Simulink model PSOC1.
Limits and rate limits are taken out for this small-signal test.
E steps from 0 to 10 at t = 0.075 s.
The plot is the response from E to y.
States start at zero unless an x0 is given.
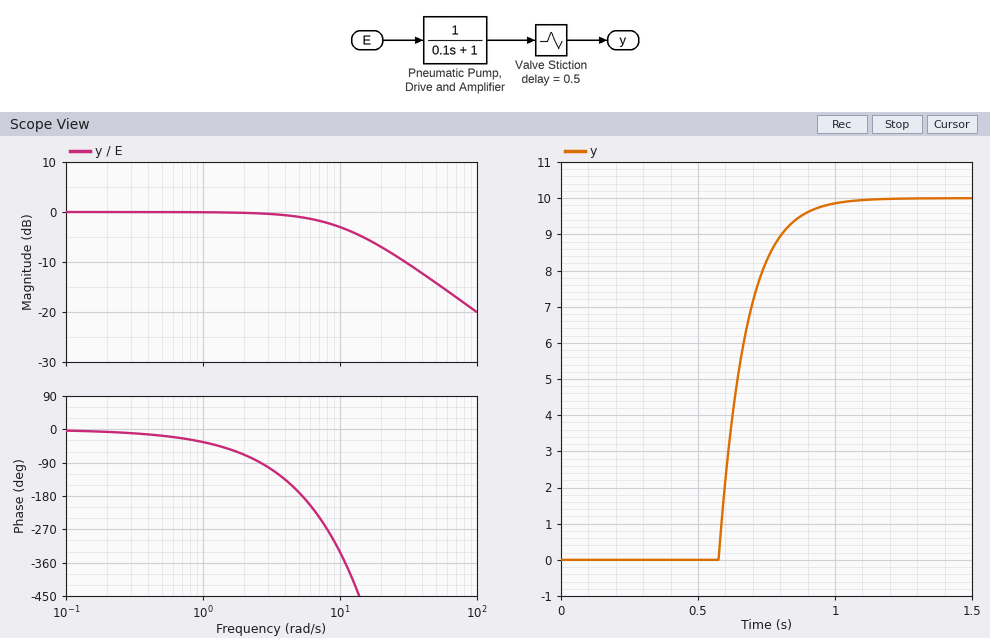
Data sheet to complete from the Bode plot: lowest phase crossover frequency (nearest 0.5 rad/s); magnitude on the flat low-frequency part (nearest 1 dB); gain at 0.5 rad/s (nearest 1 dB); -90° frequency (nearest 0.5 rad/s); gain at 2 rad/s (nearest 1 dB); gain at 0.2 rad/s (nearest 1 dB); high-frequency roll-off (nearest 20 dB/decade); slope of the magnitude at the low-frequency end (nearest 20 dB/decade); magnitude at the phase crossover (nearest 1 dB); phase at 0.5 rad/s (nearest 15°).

5.5 rad/s
0 dB
0 dB
2.5 rad/s
0 dB
0 dB
-20 dB/decade
0 dB/decade
-1 dB
-15°
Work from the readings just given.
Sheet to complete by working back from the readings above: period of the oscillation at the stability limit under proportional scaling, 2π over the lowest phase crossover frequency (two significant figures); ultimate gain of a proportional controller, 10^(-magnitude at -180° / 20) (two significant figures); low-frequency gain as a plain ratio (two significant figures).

1.1 s
1.1
1.0
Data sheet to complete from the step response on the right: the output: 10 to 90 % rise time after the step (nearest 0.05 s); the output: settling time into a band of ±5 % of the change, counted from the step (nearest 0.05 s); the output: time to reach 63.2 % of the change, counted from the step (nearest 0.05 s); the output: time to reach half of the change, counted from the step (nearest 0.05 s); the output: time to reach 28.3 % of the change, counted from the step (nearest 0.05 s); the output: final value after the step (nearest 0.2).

0.20 s
0.80 s
0.60 s
0.55 s
0.55 s
10.0
